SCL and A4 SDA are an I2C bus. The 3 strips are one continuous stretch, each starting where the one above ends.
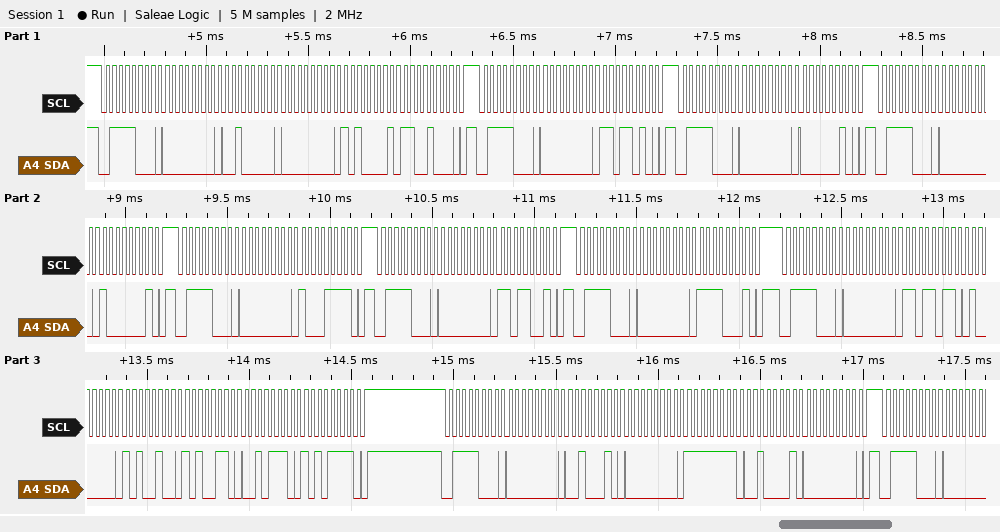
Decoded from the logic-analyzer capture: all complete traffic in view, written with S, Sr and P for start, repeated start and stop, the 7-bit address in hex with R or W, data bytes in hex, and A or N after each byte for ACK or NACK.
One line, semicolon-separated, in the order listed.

S 3CW A 00 A 20 A 00 A A1 A C8 A P S 3CW A 00 A DA A P S 3CW A 00 A 02 A P S 3CW A 00 A 81 A P S 3CW A 00 A 8F A P S 3CW A 00 A D9 A P S 3CW A 00 A F1 A P S 3CW A 00 A DB A 40 A A4 A A6 A 2E A AF A P S 3CW A 00 A 22 A 00 A FF A 21 A 00 A P S 3CW A
